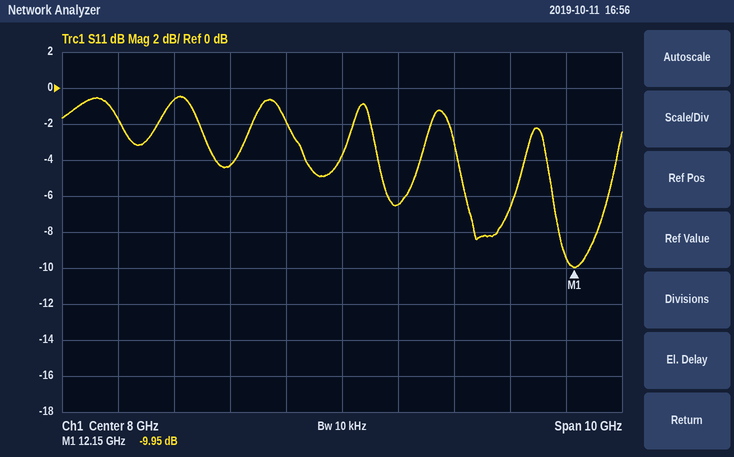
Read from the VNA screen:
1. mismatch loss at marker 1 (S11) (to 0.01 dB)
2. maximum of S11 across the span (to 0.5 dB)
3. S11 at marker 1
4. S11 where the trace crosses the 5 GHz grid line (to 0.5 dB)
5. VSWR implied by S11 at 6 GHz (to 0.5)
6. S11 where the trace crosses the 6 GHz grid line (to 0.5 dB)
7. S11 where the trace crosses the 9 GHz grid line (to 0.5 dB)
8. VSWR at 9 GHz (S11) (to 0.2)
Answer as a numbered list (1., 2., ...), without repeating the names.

1. 0.46 dB
2. -0.5 dB
3. -9.95 dB
4. -0.5 dB
5. 4.0
6. -4.5 dB
7. -6.5 dB
8. 2.8
